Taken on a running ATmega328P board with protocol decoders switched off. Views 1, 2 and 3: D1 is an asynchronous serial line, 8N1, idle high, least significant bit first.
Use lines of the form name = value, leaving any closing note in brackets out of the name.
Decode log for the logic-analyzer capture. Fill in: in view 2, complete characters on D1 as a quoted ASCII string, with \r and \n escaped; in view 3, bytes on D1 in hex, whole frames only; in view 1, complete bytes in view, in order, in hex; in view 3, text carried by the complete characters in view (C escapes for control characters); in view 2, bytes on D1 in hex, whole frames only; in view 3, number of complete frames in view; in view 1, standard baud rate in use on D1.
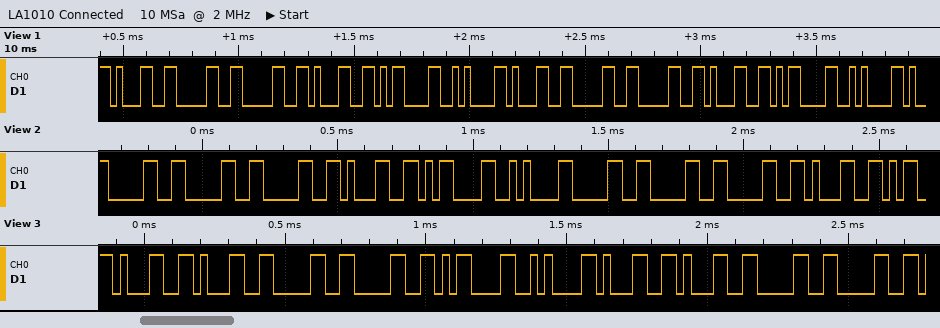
in view 2, complete characters on D1 as a quoted ASCII string, with \r and \n escaped = "0001\r\n0001"
in view 3, bytes on D1 in hex, whole frames only = 31 31 30 30 0D 0A 31 31 30 30
in view 1, complete bytes in view, in order, in hex = 31 30 30 31 0D 0A 31 30 30 31 0D 0A
in view 3, text carried by the complete characters in view = "1100\r\n1100"
in view 2, bytes on D1 in hex, whole frames only = 30 30 30 31 0D 0A 30 30 30 31
in view 3, number of complete frames in view = 10
in view 1, standard baud rate in use on D1 = 38400 baud
